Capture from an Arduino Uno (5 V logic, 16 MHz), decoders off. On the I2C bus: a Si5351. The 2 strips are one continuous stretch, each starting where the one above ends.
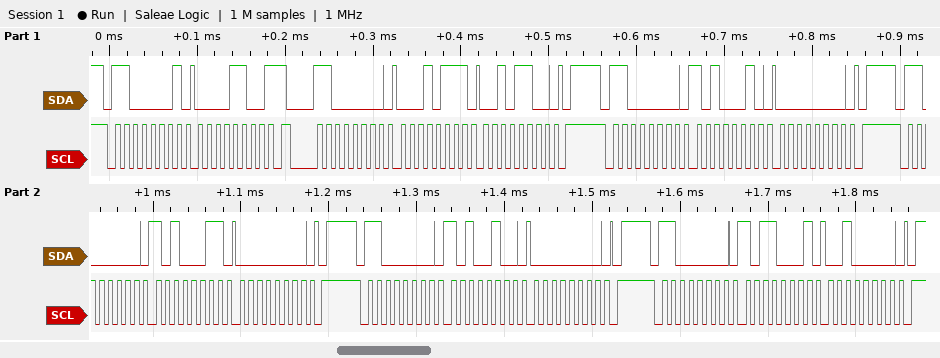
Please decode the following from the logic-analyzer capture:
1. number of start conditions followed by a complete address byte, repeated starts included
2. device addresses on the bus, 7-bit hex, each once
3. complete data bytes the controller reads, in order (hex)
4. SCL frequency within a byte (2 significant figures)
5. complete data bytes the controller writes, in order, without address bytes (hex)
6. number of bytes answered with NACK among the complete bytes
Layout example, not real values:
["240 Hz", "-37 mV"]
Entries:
["6", "0x60", "0C", "100 kHz", "17 2C A2 00 A3 00 A4 00 B1 20", "1"]
